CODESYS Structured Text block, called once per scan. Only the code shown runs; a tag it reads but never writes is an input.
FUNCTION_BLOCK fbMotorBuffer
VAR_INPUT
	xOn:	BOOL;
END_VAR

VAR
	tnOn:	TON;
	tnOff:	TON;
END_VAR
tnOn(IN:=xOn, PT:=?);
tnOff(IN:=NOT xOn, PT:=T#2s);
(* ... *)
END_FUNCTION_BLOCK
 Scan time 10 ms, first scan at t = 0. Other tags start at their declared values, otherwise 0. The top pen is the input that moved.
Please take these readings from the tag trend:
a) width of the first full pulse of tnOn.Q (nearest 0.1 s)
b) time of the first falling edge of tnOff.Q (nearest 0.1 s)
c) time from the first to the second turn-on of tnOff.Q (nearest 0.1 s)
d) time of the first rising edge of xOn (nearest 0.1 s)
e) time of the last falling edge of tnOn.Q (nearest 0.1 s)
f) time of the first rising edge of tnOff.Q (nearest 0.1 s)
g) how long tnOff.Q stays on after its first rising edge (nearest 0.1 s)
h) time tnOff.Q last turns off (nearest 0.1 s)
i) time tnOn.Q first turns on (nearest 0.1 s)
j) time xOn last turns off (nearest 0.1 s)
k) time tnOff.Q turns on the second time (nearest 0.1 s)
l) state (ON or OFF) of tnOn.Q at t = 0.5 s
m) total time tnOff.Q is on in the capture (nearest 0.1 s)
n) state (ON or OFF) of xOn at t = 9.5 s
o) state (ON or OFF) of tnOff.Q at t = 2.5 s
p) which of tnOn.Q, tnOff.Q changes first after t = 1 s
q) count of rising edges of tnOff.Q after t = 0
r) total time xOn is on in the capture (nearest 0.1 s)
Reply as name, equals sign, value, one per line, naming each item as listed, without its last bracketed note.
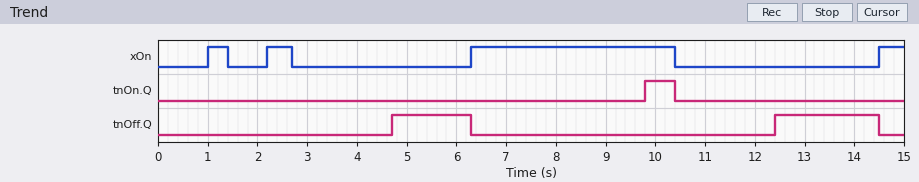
width of the first full pulse of tnOn.Q = 0.6 s
time of the first falling edge of tnOff.Q = 6.3 s
time from the first to the second turn-on of tnOff.Q = 7.7 s
time of the first rising edge of xOn = 1.0 s
time of the last falling edge of tnOn.Q = 10.4 s
time of the first rising edge of tnOff.Q = 4.7 s
how long tnOff.Q stays on after its first rising edge = 1.6 s
time tnOff.Q last turns off = 14.5 s
time tnOn.Q first turns on = 9.8 s
time xOn last turns off = 10.4 s
time tnOff.Q turns on the second time = 12.4 s
state (ON or OFF) of tnOn.Q at t = 0.5 s = OFF
total time tnOff.Q is on in the capture = 3.7 s
state (ON or OFF) of xOn at t = 9.5 s = ON
state (ON or OFF) of tnOff.Q at t = 2.5 s = OFF
which of tnOn.Q, tnOff.Q changes first after t = 1 s = tnOff.Q
count of rising edges of tnOff.Q after t = 0 = 2
total time xOn is on in the capture = 5.5 s
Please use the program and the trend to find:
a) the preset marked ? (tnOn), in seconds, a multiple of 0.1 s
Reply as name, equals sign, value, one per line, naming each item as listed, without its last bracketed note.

the preset marked ? (tnOn), in seconds, a multiple of 0.1 s = 3.5 s
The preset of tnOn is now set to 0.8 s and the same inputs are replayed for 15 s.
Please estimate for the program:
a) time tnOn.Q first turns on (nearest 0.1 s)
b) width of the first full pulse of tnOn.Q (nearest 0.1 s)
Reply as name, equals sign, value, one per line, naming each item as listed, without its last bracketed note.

time tnOn.Q first turns on = 7.1 s
width of the first full pulse of tnOn.Q = 3.3 s
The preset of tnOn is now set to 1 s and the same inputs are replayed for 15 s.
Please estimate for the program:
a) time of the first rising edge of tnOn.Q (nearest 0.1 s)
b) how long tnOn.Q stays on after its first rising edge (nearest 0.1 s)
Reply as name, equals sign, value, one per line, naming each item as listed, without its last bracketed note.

time of the first rising edge of tnOn.Q = 7.3 s
how long tnOn.Q stays on after its first rising edge = 3.1 s
